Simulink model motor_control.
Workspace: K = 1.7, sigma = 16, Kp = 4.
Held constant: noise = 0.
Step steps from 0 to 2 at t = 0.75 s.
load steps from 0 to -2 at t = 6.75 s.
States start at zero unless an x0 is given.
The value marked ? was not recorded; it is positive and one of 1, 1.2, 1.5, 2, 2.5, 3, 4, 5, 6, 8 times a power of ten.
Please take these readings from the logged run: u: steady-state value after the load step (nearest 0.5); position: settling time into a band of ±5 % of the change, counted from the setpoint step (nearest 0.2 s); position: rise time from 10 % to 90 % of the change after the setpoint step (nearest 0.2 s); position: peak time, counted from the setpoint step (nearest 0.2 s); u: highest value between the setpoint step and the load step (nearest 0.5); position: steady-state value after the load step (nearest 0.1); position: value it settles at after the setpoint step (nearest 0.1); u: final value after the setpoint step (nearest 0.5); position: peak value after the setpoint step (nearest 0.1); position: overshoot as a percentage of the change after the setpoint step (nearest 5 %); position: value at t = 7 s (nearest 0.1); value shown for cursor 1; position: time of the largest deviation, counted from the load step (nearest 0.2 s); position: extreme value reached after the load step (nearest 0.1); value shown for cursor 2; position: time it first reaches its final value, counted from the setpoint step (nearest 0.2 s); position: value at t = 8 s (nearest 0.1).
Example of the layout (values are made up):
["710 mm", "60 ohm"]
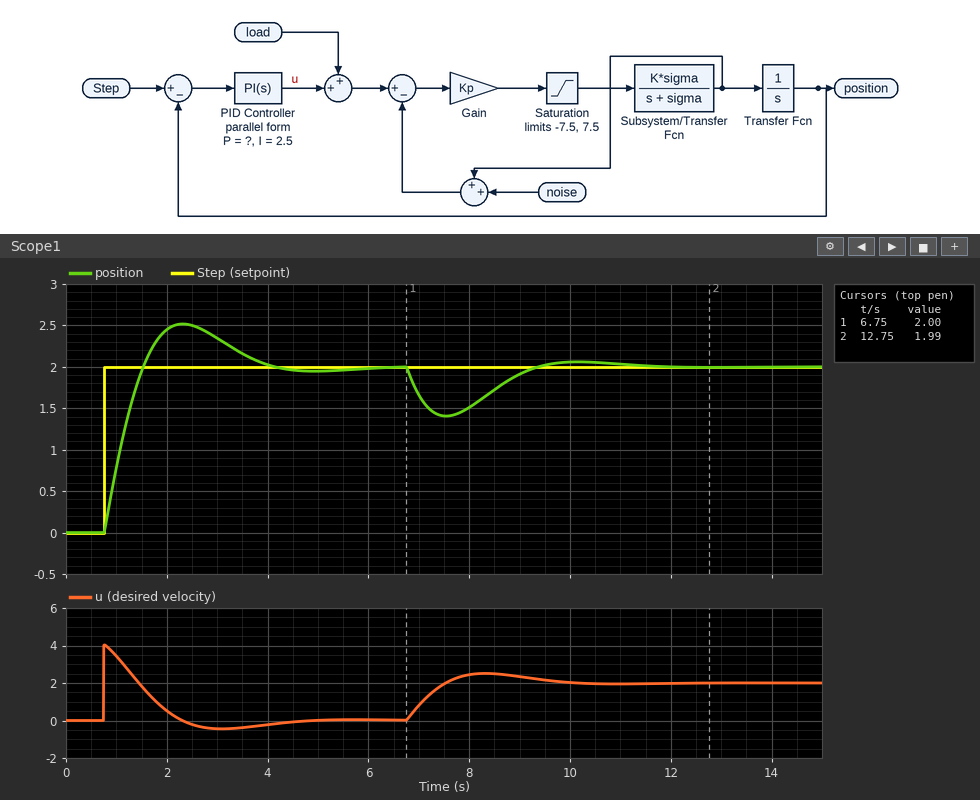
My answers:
["2.0", "3.0 s", "0.6 s", "1.6 s", "4.0", "2.0", "2.0", "0.0", "2.5", "25 %", "1.7", "2.00", "0.8 s", "1.4", "1.99", "0.8 s", "1.5"]
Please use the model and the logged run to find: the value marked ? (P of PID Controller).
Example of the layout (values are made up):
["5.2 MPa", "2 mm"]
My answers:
["2"]
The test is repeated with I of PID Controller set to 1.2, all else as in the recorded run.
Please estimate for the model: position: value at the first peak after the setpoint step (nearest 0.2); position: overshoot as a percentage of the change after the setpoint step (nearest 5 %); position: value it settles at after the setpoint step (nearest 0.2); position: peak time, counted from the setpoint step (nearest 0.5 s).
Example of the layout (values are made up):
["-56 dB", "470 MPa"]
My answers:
["2.4", "15 %", "2.0", "2.0 s"]
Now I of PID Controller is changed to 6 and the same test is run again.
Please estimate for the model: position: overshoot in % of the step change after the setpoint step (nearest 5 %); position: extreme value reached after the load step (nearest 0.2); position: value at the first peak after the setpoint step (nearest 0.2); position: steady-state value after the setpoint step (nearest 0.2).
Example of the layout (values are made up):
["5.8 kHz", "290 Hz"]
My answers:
["40 %", "1.6", "2.8", "2.0"]
